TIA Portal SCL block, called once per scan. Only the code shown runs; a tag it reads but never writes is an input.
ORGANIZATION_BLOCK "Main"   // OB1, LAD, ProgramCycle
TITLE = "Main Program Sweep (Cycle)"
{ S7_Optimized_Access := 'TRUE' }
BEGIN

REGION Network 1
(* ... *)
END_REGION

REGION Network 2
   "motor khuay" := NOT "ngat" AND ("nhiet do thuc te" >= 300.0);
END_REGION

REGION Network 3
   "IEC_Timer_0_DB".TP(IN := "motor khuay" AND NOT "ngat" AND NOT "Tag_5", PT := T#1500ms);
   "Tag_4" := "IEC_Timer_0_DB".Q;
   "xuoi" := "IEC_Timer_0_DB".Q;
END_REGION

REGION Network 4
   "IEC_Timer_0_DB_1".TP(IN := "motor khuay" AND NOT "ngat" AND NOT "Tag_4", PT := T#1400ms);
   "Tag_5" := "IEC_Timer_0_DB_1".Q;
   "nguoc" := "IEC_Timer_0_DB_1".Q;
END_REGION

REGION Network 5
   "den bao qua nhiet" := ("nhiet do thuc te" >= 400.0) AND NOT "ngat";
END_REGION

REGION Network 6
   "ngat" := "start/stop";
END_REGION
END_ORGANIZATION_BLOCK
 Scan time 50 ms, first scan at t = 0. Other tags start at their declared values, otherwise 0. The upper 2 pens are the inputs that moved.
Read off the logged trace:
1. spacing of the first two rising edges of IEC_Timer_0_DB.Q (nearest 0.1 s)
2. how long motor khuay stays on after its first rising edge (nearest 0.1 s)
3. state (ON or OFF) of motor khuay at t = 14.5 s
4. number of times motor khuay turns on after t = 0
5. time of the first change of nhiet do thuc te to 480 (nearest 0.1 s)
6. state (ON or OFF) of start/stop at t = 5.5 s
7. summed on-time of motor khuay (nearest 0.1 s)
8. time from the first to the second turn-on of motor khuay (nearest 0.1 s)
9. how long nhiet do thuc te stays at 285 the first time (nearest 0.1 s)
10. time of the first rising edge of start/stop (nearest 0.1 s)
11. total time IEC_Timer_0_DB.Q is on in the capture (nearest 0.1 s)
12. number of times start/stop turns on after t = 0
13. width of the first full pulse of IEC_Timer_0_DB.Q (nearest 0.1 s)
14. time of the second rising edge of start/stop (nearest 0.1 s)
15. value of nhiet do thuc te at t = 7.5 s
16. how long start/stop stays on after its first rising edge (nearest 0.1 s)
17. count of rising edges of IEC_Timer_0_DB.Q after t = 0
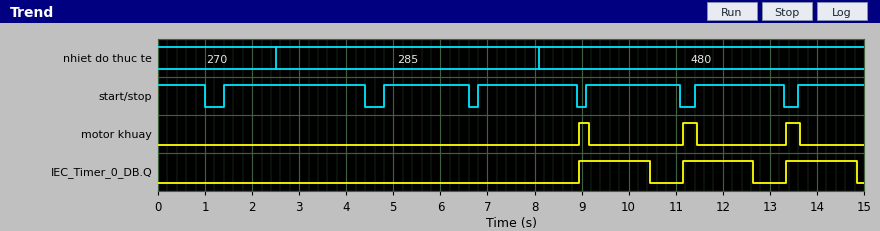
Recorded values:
2.2 s
0.2 s
OFF
3
8.1 s
ON
0.8 s
2.2 s
5.6 s
1.4 s
4.5 s
6
1.5 s
4.8 s
285
3.0 s
3
